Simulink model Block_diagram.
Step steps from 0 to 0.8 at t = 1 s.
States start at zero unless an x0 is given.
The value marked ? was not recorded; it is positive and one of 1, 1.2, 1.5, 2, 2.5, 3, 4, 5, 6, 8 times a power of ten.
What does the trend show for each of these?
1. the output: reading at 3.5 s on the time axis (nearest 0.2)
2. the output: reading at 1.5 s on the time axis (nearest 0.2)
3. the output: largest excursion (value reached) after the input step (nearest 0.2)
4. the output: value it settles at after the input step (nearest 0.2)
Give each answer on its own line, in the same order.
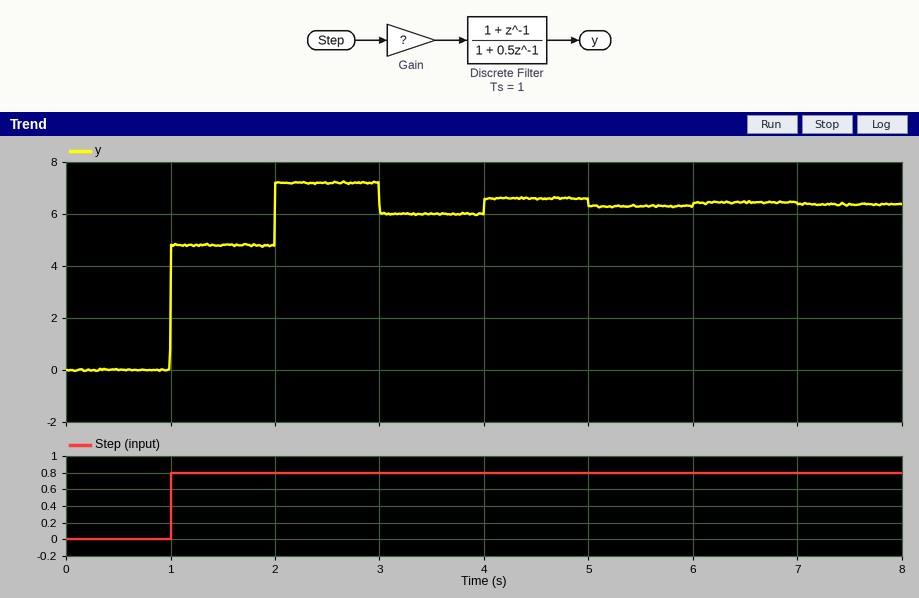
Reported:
6.0
4.8
7.2
6.4
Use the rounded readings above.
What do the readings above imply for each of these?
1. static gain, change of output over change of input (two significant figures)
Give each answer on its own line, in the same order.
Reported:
8.0
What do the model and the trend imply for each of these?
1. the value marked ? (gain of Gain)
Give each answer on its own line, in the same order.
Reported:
6
